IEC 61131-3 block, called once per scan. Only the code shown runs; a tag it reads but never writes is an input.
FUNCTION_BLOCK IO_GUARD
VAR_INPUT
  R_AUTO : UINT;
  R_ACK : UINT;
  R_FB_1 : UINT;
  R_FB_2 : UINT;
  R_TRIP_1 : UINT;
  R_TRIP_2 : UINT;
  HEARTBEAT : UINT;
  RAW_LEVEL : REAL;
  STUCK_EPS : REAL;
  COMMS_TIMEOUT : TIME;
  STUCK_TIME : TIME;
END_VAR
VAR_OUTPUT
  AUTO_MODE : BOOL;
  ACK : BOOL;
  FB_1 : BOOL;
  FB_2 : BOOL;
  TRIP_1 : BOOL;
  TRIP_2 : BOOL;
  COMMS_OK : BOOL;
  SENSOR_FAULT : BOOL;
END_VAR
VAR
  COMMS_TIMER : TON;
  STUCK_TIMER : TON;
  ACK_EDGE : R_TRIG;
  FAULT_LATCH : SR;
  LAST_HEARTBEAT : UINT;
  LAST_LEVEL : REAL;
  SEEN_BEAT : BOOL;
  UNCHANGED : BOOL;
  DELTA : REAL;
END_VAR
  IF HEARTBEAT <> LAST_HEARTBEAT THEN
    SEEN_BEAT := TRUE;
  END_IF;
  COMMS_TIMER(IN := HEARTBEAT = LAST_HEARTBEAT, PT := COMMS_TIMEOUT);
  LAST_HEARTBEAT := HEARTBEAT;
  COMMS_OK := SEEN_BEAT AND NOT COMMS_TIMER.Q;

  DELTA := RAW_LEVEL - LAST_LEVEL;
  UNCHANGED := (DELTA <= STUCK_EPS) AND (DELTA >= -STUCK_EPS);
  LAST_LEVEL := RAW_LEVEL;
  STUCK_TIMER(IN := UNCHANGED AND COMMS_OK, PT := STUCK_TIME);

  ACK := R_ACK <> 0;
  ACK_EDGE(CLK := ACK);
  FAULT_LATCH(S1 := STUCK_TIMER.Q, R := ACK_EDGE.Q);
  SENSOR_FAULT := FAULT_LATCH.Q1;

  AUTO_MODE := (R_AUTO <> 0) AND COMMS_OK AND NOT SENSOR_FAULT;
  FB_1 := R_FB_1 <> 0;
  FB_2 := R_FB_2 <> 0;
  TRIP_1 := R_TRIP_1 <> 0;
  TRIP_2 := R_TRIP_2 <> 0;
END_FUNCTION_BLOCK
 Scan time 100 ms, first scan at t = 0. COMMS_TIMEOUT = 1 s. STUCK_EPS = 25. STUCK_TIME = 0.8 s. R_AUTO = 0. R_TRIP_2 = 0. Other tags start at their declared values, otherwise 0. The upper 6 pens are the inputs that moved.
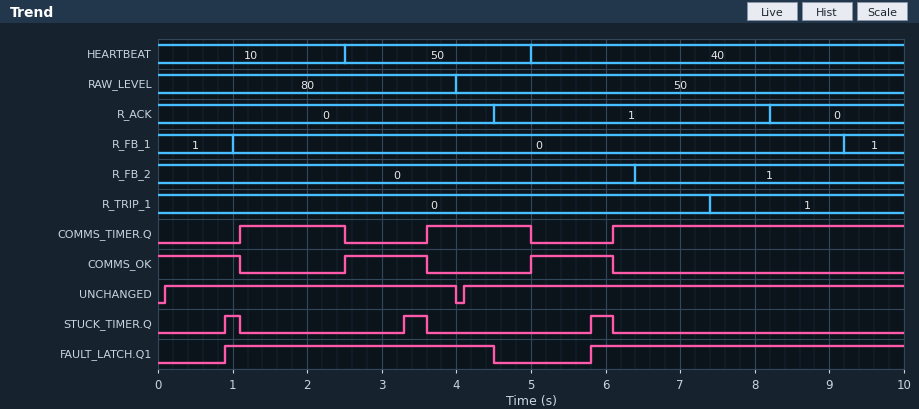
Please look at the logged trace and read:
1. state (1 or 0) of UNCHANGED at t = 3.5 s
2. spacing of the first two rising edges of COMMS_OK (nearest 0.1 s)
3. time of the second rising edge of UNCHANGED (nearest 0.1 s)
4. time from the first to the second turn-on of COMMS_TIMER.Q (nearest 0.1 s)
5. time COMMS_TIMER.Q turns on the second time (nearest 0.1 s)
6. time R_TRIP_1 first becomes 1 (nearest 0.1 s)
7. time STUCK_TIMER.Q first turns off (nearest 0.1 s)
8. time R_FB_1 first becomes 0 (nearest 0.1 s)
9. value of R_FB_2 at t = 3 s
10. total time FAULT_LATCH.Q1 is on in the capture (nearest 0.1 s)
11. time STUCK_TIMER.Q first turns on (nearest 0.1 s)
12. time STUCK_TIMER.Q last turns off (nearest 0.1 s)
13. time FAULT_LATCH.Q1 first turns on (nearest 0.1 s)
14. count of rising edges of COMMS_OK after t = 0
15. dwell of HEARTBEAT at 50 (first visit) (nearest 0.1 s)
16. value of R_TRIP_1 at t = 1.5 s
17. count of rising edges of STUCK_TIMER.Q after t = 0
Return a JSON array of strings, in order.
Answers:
["1", "2.5 s", "4.1 s", "2.5 s", "3.6 s", "7.4 s", "1.1 s", "1.0 s", "0", "7.8 s", "0.9 s", "6.1 s", "0.9 s", "2", "2.5 s", "0", "3"]
